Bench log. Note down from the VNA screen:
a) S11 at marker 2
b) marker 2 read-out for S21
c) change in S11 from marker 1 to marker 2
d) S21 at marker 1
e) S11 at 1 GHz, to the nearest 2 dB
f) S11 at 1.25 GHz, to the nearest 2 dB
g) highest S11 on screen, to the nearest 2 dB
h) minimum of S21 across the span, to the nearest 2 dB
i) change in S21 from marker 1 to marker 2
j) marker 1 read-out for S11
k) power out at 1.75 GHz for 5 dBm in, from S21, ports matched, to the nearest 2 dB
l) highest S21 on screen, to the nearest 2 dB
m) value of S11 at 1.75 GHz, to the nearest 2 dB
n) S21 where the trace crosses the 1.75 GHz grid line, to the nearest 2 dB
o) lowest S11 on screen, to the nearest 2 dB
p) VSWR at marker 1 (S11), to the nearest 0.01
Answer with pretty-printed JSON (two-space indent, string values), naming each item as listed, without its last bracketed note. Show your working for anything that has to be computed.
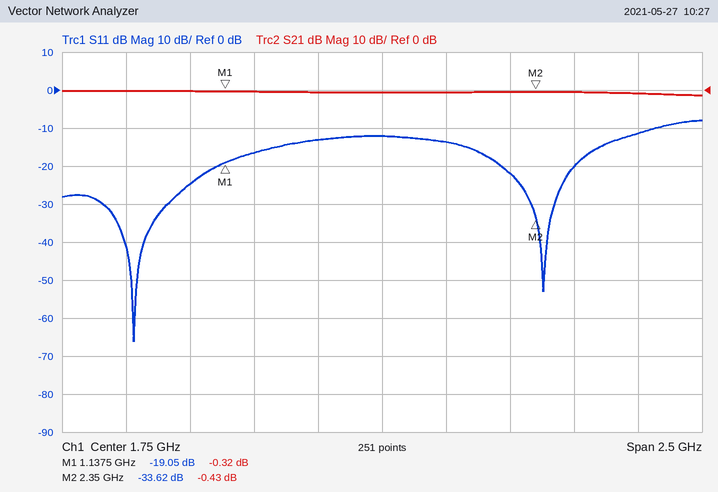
{
  "S11 at marker 2": "-33.62 dB",
  "marker 2 read-out for S21": "-0.43 dB",
  "change in S11 from marker 1 to marker 2": "-33.62 − (-19.05) = -14.57 dB",
  "S21 at marker 1": "-0.32 dB",
  "S11 at 1 GHz, to the nearest 2 dB": "-24 dB",
  "S11 at 1.25 GHz, to the nearest 2 dB": "-16 dB",
  "highest S11 on screen, to the nearest 2 dB": "-8 dB",
  "minimum of S21 across the span, to the nearest 2 dB": "-2 dB",
  "change in S21 from marker 1 to marker 2": "-0.43 − (-0.32) = -0.11 dB",
  "marker 1 read-out for S11": "-19.05 dB",
  "power out at 1.75 GHz for 5 dBm in, from S21, ports matched, to the nearest 2 dB": "5 dBm + (0 dB) = 4 dBm",
  "highest S21 on screen, to the nearest 2 dB": "0 dB",
  "value of S11 at 1.75 GHz, to the nearest 2 dB": "-12 dB",
  "S21 where the trace crosses the 1.75 GHz grid line, to the nearest 2 dB": "0 dB",
  "lowest S11 on screen, to the nearest 2 dB": "-66 dB",
  "VSWR at marker 1 (S11), to the nearest 0.01": "(1 + 0.1116)/(1 − 0.1116) ≈ 1.25"
}
